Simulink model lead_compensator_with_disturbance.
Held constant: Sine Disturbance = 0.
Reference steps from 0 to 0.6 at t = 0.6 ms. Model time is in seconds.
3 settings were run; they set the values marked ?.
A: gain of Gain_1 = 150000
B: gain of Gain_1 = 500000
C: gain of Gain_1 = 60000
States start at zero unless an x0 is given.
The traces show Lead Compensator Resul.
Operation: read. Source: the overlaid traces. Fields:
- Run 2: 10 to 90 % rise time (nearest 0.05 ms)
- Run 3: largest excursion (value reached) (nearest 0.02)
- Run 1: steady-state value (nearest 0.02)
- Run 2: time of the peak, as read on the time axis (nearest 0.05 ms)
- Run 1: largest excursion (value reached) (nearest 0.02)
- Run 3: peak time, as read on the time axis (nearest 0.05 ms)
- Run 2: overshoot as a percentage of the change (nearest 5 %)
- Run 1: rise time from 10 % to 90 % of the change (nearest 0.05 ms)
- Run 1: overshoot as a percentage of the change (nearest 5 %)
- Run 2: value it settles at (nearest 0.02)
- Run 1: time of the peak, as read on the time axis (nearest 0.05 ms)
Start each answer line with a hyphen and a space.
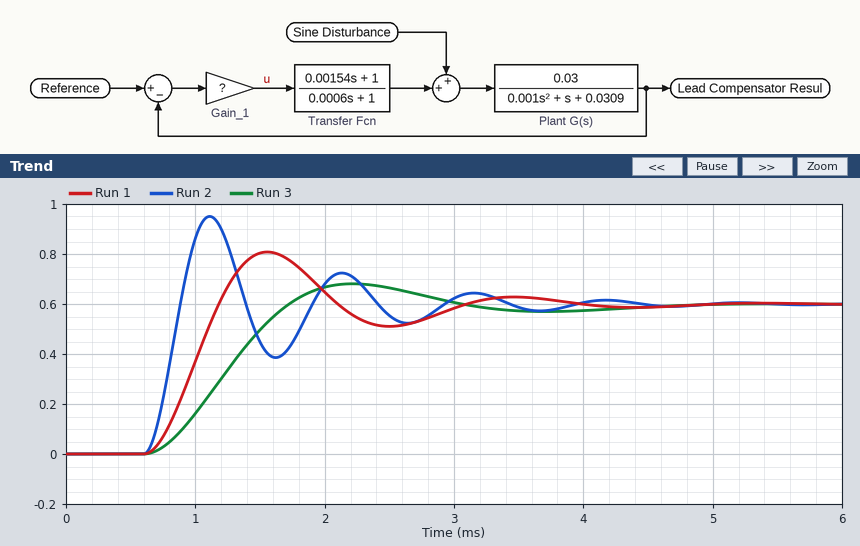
- 0.20 ms
- 0.68
- 0.60
- 1.10 ms
- 0.80
- 2.20 ms
- 60 %
- 0.40 ms
- 35 %
- 0.60
- 1.55 ms
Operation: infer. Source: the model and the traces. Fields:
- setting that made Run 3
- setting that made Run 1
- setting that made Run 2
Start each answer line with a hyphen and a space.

- C
- A
- B
